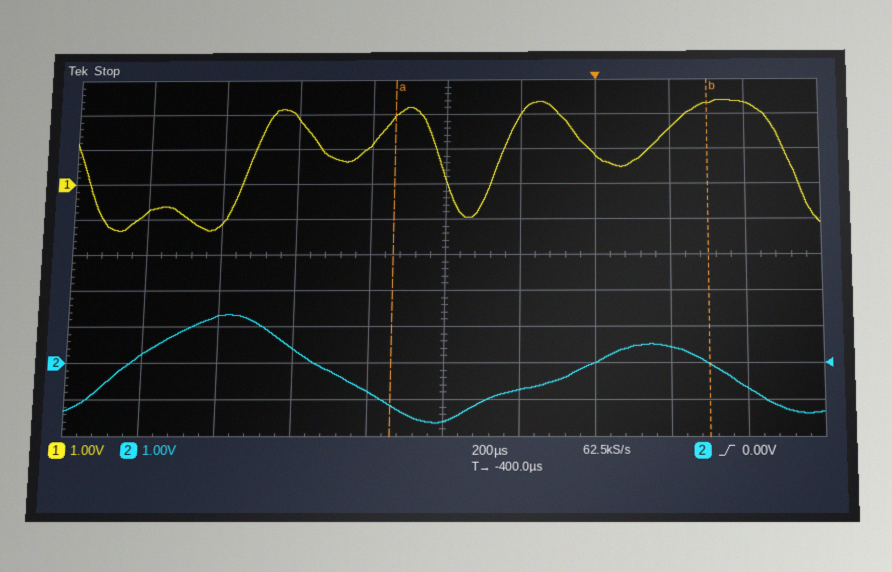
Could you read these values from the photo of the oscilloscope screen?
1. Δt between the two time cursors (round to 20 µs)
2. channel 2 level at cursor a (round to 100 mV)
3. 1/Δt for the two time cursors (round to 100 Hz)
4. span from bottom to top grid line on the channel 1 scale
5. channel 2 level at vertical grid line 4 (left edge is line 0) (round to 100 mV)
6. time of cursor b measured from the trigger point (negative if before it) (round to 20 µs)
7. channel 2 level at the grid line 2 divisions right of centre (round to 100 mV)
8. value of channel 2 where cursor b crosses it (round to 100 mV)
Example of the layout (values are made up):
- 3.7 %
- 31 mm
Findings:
- 840 µs
- -1.2 V
- 1.2 kHz
- 10 V
- -800 mV
- +300 µs
- 0.0 V
- 0.0 V
